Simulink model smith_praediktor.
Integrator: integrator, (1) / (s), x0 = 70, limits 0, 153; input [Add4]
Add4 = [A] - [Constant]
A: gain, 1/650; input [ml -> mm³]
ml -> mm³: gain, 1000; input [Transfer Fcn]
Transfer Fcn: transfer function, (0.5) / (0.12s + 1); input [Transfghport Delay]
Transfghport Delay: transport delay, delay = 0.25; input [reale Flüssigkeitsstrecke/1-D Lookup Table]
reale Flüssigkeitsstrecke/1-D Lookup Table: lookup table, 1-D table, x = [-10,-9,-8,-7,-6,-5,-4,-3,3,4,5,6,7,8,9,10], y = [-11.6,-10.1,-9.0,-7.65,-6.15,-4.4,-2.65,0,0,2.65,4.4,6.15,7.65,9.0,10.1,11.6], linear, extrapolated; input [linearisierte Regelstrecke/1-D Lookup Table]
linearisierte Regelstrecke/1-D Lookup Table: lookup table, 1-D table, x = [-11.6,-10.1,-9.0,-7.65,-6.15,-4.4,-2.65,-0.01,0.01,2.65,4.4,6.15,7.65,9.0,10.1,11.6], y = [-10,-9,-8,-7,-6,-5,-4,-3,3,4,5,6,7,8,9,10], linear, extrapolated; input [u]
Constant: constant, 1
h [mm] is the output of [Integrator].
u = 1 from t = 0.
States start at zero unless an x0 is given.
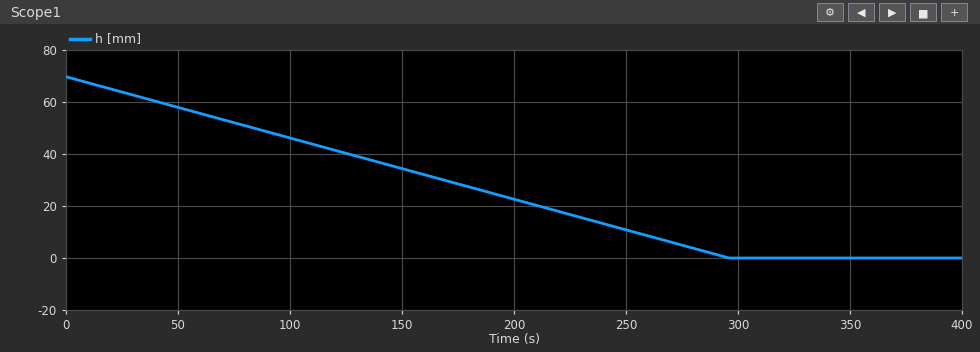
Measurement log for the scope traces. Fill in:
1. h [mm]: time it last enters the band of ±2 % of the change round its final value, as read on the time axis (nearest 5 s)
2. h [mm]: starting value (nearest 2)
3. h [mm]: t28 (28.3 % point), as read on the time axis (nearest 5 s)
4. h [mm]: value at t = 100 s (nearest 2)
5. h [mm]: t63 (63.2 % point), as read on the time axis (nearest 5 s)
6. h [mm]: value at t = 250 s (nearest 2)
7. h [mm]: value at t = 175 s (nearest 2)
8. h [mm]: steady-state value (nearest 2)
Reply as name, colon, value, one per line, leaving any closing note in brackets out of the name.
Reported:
h [mm]: time it last enters the band of ±2 % of the change round its final value, as read on the time axis: 290 s
h [mm]: starting value: 70
h [mm]: t28 (28.3 % point), as read on the time axis: 85 s
h [mm]: value at t = 100 s: 46
h [mm]: t63 (63.2 % point), as read on the time axis: 185 s
h [mm]: value at t = 250 s: 10
h [mm]: value at t = 175 s: 28
h [mm]: steady-state value: 0
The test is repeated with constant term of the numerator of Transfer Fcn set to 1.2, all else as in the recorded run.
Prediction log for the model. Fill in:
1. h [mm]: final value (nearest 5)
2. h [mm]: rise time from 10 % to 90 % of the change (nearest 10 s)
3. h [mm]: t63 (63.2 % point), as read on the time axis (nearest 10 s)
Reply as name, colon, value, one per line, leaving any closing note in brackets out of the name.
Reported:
h [mm]: final value: 155
h [mm]: rise time from 10 % to 90 % of the change: 80 s
h [mm]: t63 (63.2 % point), as read on the time axis: 60 s
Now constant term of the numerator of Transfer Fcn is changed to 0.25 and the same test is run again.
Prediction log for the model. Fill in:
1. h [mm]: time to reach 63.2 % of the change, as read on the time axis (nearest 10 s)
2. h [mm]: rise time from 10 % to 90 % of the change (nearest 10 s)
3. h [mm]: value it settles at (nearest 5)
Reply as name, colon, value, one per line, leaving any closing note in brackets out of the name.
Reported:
h [mm]: time to reach 63.2 % of the change, as read on the time axis: 70 s
h [mm]: rise time from 10 % to 90 % of the change: 90 s
h [mm]: value it settles at: 0
